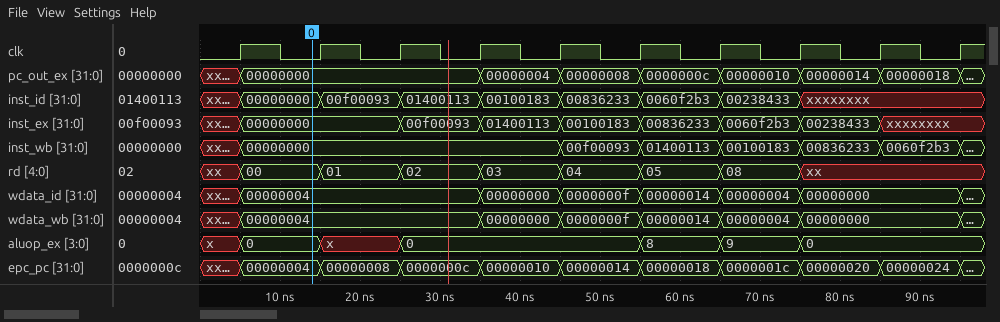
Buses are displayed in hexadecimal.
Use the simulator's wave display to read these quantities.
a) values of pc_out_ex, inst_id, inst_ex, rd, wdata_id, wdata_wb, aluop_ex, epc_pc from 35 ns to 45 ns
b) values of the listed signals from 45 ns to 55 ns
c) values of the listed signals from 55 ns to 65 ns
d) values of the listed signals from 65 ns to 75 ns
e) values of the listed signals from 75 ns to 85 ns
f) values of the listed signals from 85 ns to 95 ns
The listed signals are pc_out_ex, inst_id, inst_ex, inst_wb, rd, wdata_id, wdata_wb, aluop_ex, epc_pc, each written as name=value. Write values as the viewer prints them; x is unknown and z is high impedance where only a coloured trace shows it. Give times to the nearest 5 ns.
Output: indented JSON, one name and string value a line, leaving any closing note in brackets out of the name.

{
  "values of pc_out_ex, inst_id, inst_ex, rd, wdata_id, wdata_wb, aluop_ex, epc_pc from 35 ns to 45 ns": "pc_out_ex=00000004, inst_id=00100183, inst_ex=01400113, rd=03, wdata_id=00000000, wdata_wb=00000000, aluop_ex=0, epc_pc=00000010",
  "values of the listed signals from 45 ns to 55 ns": "pc_out_ex=00000008, inst_id=00836233, inst_ex=00100183, inst_wb=00f00093, rd=04, wdata_id=0000000f, wdata_wb=0000000f, aluop_ex=0, epc_pc=00000014",
  "values of the listed signals from 55 ns to 65 ns": "pc_out_ex=0000000c, inst_id=0060f2b3, inst_ex=00836233, inst_wb=01400113, rd=05, wdata_id=00000014, wdata_wb=00000014, aluop_ex=8, epc_pc=00000018",
  "values of the listed signals from 65 ns to 75 ns": "pc_out_ex=00000010, inst_id=00238433, inst_ex=0060f2b3, inst_wb=00100183, rd=08, wdata_id=00000004, wdata_wb=00000004, aluop_ex=9, epc_pc=0000001c",
  "values of the listed signals from 75 ns to 85 ns": "pc_out_ex=00000014, inst_id=xxxxxxxx, inst_ex=00238433, inst_wb=00836233, rd=xx, wdata_id=00000000, wdata_wb=00000000, aluop_ex=0, epc_pc=00000020",
  "values of the listed signals from 85 ns to 95 ns": "pc_out_ex=00000018, inst_id=xxxxxxxx, inst_ex=xxxxxxxx, inst_wb=0060f2b3, rd=xx, wdata_id=00000000, wdata_wb=00000000, aluop_ex=0, epc_pc=00000024"
}
